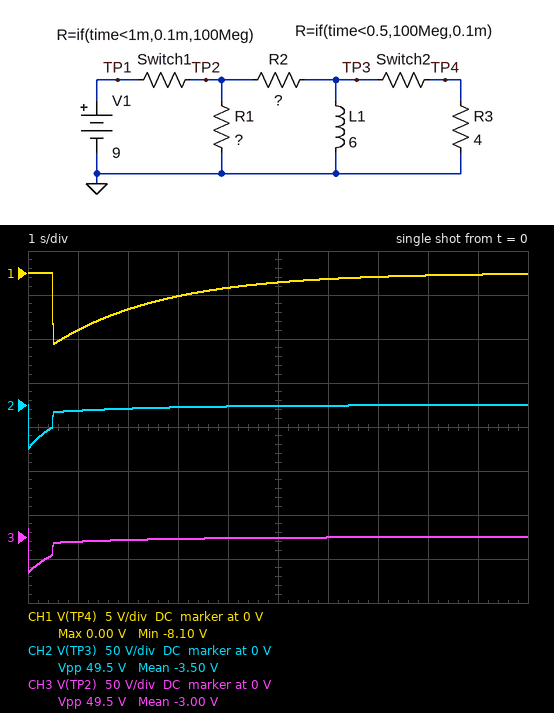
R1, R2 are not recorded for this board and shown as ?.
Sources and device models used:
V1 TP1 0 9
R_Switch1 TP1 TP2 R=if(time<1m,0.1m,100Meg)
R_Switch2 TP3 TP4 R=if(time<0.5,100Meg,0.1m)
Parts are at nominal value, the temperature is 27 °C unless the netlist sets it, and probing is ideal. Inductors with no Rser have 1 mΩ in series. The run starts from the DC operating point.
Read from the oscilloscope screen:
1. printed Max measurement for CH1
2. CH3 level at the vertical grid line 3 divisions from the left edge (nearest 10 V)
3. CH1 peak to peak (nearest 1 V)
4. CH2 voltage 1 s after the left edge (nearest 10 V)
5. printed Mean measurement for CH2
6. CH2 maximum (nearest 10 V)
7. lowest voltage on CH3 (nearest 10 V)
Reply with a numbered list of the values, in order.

1. 0.00 V
2. 0 V
3. 8 V
4. -10 V
5. -3.50 V
6. 0 V
7. -40 V
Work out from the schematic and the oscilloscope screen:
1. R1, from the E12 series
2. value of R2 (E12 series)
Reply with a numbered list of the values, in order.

1. 6.8 Ω
2. 1.5 Ω
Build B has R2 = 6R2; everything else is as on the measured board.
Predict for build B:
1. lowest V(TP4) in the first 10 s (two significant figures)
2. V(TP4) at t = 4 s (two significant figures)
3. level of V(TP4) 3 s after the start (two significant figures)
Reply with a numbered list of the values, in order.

1. -1.5 V
2. -250 mV
3. -420 mV
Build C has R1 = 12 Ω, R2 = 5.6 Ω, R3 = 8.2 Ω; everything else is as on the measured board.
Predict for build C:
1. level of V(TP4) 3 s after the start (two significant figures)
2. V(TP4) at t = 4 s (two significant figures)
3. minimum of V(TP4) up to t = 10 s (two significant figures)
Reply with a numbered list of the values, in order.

1. -200 mV
2. -80 mV
3. -2.1 V
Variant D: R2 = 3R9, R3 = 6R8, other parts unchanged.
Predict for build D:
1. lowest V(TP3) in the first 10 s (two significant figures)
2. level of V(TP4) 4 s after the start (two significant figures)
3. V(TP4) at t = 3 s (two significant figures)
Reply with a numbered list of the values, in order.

1. -25 V
2. -350 mV
3. -700 mV
